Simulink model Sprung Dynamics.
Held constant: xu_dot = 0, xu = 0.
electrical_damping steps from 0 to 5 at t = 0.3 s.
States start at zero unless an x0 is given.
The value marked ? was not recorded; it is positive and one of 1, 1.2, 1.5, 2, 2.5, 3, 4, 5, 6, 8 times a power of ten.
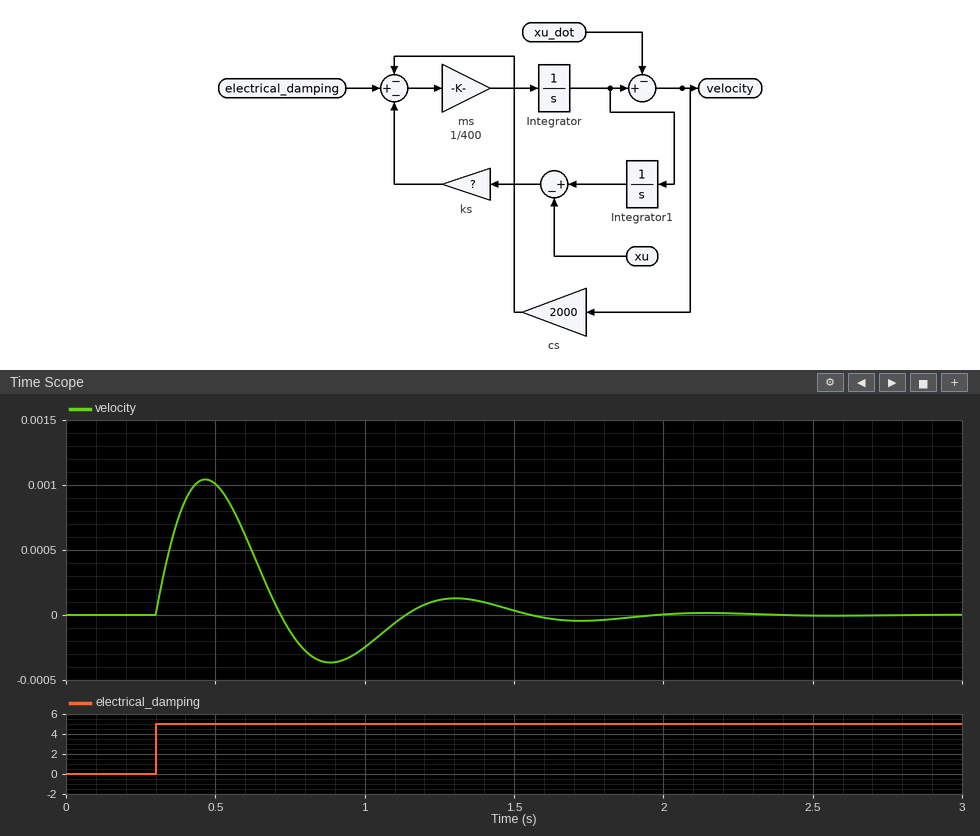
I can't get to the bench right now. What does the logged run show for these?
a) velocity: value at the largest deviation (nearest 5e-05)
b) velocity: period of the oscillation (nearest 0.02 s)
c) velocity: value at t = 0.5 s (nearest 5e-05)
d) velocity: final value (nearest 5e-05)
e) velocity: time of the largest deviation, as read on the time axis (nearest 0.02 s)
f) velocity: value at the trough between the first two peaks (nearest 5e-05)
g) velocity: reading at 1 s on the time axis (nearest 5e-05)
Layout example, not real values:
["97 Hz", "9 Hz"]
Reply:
["0.00105", "0.84 s", "0.00100", "0.00000", "0.46 s", "-0.00035", "-0.00025"]
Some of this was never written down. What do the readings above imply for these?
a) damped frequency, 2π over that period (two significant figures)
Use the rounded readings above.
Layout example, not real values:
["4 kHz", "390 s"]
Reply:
["7.5 rad/s"]
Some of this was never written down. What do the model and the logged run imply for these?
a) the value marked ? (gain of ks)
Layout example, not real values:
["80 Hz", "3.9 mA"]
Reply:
["25000"]
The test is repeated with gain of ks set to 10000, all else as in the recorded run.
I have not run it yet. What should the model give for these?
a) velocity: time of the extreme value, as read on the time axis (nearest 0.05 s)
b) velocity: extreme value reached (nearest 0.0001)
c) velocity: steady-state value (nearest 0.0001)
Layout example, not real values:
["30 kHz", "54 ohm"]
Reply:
["0.55 s", "0.0014", "0.0000"]
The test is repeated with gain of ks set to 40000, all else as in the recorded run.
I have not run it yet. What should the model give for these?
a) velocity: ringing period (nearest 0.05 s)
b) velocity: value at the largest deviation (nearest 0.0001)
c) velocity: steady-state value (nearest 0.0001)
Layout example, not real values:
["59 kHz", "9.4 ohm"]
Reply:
["0.65 s", "0.0009", "0.0000"]
